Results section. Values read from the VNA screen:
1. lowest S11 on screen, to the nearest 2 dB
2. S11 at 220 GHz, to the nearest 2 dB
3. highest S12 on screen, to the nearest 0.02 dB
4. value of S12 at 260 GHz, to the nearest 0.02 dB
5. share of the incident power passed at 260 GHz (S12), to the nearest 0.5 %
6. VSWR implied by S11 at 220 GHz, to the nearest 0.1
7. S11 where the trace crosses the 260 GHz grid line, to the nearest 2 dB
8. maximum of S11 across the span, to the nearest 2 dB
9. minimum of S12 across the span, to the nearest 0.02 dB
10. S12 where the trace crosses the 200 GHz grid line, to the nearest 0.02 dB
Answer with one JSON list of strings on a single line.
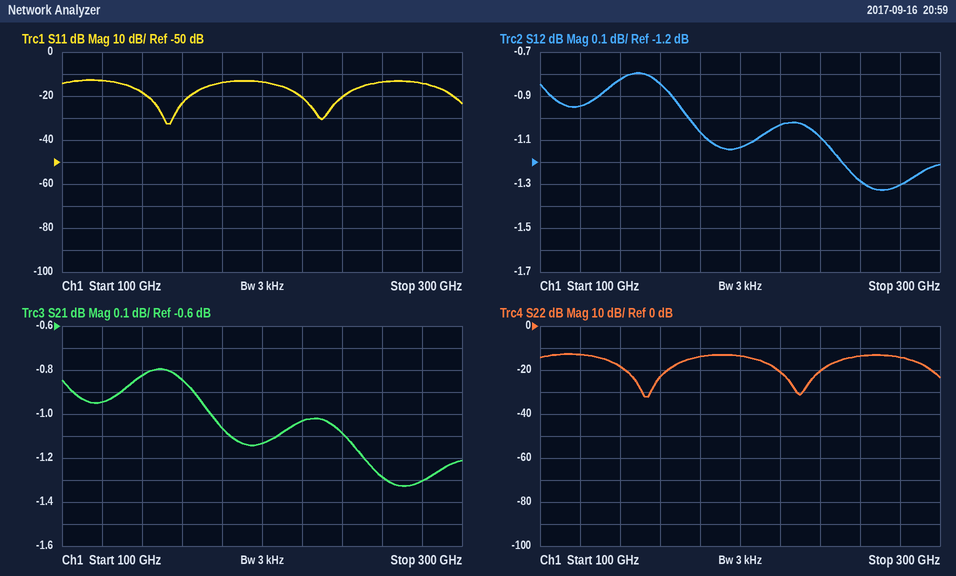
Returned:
["-32 dB", "-20 dB", "-0.80 dB", "-1.28 dB", "74.5 %", "1.2", "-14 dB", "-12 dB", "-1.32 dB", "-1.14 dB"]
